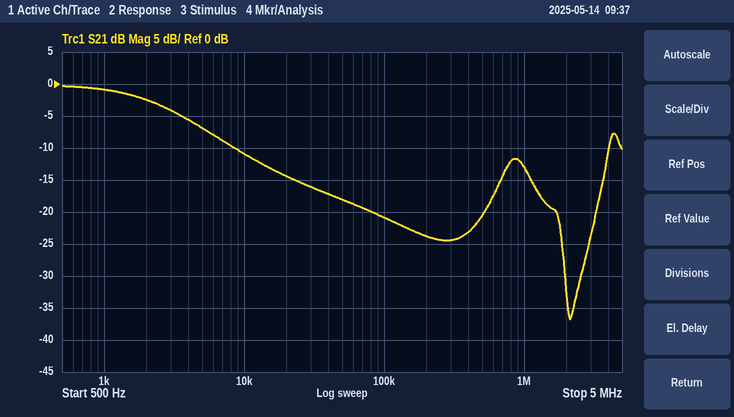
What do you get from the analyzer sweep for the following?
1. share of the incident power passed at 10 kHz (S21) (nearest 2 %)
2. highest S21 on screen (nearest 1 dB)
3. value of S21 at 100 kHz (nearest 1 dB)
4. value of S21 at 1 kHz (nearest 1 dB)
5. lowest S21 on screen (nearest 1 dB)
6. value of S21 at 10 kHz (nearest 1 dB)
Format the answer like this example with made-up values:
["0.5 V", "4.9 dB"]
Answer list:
["8 %", "0 dB", "-21 dB", "-1 dB", "-37 dB", "-11 dB"]
